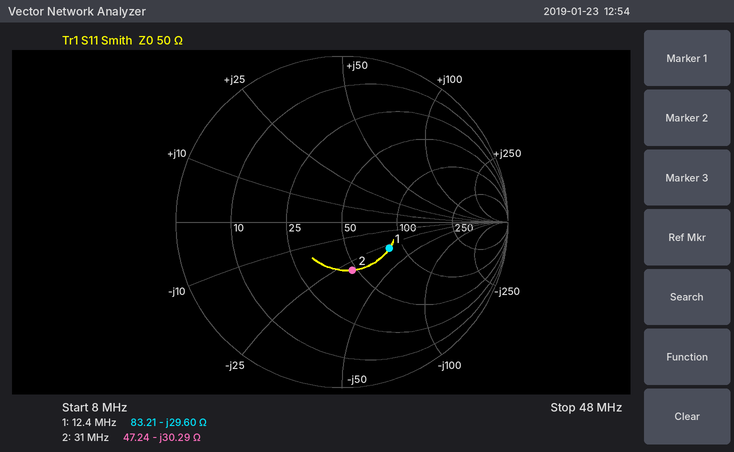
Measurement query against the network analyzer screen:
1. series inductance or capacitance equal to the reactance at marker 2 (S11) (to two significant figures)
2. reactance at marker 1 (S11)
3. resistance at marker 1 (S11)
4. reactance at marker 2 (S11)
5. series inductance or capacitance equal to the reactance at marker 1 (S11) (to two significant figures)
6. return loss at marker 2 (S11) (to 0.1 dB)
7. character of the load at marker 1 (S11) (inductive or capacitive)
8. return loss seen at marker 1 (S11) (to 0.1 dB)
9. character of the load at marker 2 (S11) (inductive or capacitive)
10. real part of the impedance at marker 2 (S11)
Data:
170 pF
-29.60 Ω
83.21 Ω
-30.29 Ω
430 pF
10.5 dB
capacitive
9.7 dB
capacitive
47.24 Ω
